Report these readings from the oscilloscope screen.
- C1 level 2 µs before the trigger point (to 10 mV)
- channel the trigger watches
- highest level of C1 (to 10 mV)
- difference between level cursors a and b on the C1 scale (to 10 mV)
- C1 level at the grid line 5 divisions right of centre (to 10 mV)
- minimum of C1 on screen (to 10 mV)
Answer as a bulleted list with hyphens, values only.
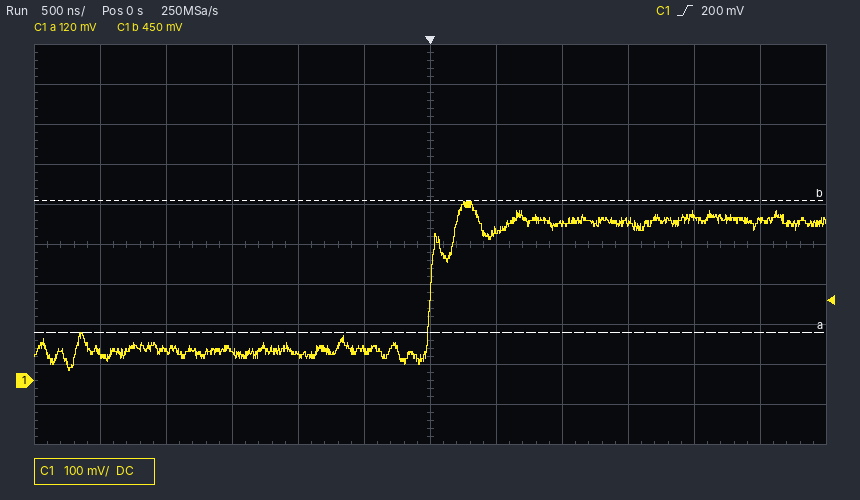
- 70 mV
- C1
- 450 mV
- 330 mV
- 400 mV
- 20 mV
